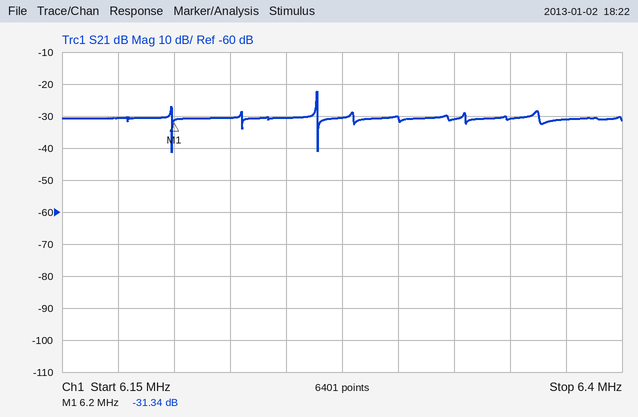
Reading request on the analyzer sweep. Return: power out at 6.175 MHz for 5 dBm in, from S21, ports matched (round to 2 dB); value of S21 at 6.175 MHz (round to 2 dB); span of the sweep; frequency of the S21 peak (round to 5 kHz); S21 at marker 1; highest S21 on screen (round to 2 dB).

-26 dBm
-30 dB
250 kHz
6.265 MHz
-31.34 dB
-22 dB
